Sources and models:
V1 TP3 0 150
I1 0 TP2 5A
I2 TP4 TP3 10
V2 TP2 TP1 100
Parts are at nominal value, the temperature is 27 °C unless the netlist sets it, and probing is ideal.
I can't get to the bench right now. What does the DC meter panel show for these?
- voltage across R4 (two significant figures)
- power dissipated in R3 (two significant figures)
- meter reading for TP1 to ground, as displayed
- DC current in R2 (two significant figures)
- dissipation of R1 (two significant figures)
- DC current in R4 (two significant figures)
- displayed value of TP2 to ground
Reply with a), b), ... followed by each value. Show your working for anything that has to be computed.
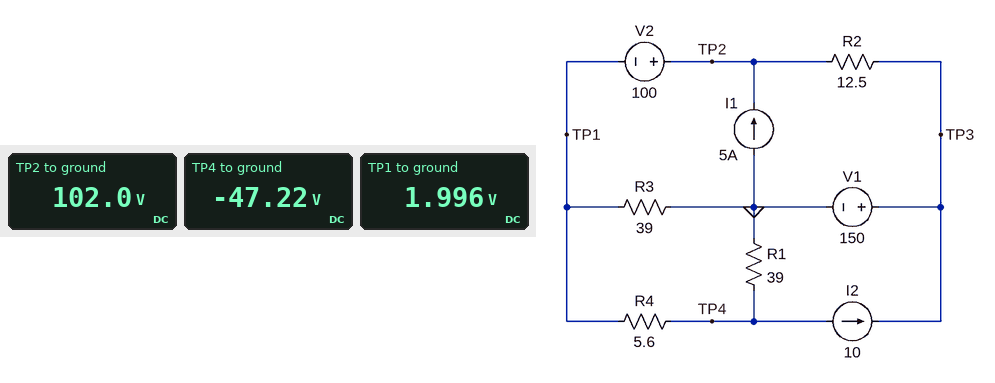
a) 1.996 V - (-47.22 V) = 49 V
b) (1.996 V)^2 / 39 Ω = 100 mW
c) 1.996 V
d) (150 V - 102 V) / 12.5 Ω = 3.8 A
e) (0 V - (-47.22 V))^2 / 39 Ω = 57 W
f) (1.996 V - (-47.22 V)) / 5.6 Ω = 8.8 A
g) 102.0 V
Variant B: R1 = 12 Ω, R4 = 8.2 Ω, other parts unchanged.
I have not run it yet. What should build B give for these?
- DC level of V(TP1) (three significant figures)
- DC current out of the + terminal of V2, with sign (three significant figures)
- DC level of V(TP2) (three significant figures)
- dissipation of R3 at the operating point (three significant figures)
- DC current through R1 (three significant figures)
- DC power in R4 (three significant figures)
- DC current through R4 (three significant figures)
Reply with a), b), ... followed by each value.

a) 19.7 V
b) -7.42 A
c) 120 V
d) 9.97 W
e) 3.08 A
f) 392 W
g) 6.92 A
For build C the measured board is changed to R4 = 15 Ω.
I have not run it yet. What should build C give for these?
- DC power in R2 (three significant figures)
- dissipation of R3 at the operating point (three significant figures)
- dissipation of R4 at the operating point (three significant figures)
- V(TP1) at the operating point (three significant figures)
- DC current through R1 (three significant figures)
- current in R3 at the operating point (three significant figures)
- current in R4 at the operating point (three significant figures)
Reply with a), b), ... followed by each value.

a) 102 W
b) 5.26 W
c) 841 W
d) 14.3 V
e) 2.51 A
f) 367 mA
g) 7.49 A
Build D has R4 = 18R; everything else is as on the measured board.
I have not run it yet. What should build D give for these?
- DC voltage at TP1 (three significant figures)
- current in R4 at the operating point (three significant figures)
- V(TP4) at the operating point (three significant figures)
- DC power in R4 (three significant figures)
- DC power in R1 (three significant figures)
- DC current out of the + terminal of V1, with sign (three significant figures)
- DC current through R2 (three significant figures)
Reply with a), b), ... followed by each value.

a) 17.5 V
b) 7.15 A
c) -111 V
d) 920 W
e) 317 W
f) -7.40 A
g) 2.60 A
